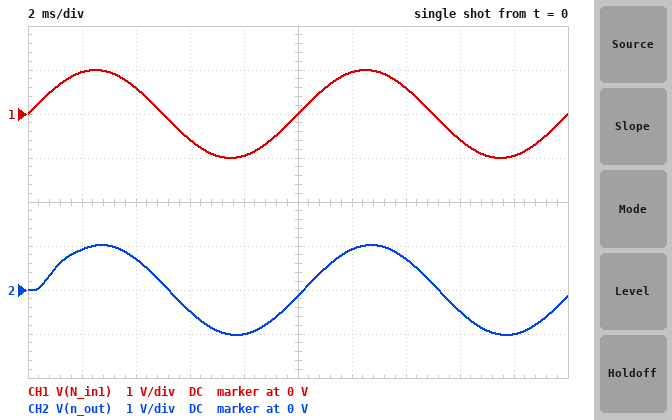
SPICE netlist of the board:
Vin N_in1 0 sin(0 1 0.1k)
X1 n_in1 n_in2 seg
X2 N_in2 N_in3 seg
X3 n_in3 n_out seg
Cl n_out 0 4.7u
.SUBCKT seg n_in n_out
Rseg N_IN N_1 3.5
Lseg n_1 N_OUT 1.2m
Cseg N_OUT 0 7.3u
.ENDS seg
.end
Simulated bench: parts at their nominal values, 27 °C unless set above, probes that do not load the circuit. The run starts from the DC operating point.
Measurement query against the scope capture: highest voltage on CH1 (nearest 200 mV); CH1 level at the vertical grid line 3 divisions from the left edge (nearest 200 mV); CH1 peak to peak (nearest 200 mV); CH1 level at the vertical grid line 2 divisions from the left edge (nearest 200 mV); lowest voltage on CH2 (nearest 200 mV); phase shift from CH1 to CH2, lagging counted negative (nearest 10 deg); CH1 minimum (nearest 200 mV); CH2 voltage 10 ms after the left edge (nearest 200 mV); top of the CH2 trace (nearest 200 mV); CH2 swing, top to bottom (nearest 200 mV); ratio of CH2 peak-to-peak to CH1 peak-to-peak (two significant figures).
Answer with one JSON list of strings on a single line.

["1.0 V", "-600 mV", "2.0 V", "600 mV", "-1.0 V", "-10 deg", "-1.0 V", "-200 mV", "1.0 V", "2.0 V", "1.0"]
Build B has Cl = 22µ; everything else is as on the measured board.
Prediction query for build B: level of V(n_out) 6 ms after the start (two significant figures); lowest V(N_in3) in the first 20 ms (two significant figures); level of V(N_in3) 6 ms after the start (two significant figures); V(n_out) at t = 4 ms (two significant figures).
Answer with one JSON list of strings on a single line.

["-380 mV", "-1.0 V", "-440 mV", "790 mV"]
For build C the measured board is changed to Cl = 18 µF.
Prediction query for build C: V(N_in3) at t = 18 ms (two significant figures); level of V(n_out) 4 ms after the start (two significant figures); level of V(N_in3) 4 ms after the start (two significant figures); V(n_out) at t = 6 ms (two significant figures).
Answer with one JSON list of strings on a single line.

["-1.0 V", "770 mV", "720 mV", "-410 mV"]
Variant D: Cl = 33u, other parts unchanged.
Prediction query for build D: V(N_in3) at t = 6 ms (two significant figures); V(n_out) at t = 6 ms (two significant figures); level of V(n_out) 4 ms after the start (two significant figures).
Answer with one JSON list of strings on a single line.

["-390 mV", "-310 mV", "830 mV"]
